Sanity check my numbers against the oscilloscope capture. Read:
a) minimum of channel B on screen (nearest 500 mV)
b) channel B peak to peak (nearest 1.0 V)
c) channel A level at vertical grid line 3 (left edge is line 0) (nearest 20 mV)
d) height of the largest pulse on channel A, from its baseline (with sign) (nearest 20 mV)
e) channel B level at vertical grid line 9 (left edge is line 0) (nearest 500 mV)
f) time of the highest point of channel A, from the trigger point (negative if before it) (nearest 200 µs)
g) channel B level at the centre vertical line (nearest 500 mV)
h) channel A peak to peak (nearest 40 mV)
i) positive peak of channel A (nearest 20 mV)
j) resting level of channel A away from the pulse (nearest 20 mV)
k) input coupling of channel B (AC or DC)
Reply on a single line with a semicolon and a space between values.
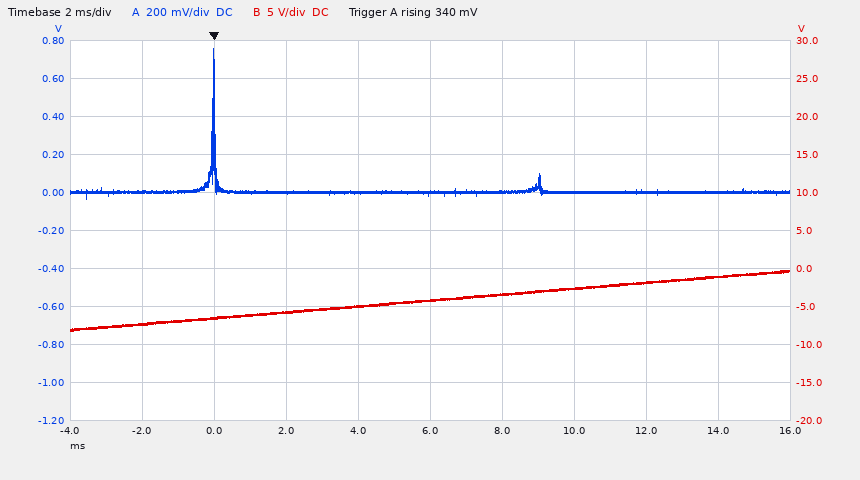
-8.0 V; 8.0 V; 0 mV; +760 mV; -1.0 V; 0.0 ms; -4.0 V; 800 mV; 760 mV; 0 mV; DC
